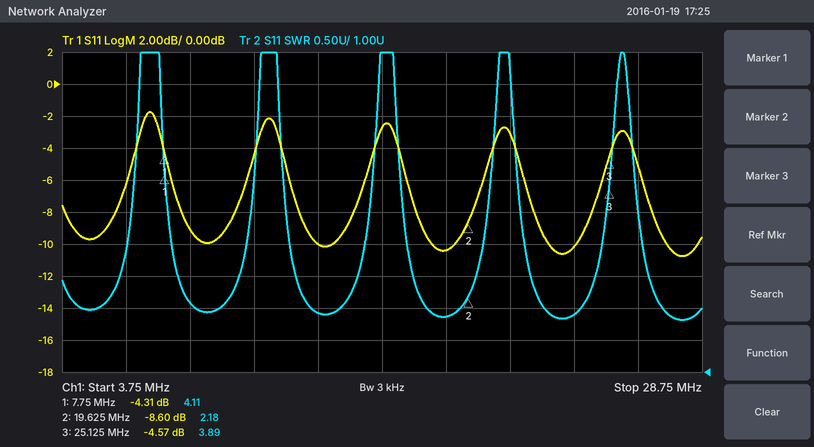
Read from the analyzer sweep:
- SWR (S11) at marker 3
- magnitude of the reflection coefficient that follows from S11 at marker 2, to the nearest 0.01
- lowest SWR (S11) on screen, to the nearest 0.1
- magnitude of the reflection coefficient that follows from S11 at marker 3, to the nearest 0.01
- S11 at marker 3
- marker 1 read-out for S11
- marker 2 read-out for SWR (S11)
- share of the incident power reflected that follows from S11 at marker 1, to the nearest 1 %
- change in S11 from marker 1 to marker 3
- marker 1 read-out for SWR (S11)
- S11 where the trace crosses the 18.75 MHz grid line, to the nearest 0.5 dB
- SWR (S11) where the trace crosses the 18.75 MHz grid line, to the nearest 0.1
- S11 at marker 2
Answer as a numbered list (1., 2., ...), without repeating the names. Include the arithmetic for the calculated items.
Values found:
1. 3.89
2. 10^(-8.6/20) ≈ 0.37
3. 1.8
4. 10^(-4.57/20) ≈ 0.59
5. -4.57 dB
6. -4.31 dB
7. 2.18
8. 10^(-4.31/10) ≈ 37 %
9. -4.57 − (-4.31) = -0.26 dB
10. 4.11
11. -10.5 dB
12. 1.9
13. -8.60 dB
